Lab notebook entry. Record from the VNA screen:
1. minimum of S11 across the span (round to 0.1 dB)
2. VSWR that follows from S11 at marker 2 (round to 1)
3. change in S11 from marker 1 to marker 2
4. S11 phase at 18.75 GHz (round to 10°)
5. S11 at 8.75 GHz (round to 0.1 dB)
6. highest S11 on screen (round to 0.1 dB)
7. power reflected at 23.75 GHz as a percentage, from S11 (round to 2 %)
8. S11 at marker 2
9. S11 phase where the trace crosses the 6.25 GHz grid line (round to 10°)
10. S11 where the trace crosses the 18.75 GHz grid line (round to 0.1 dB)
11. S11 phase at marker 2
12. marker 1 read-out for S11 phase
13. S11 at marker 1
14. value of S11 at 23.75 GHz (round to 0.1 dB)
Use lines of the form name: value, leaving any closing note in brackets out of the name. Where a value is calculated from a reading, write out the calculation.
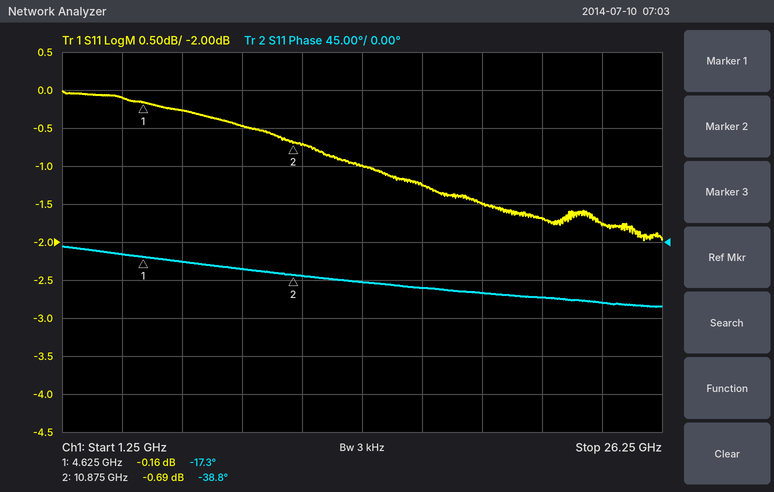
minimum of S11 across the span: -2.0 dB
VSWR that follows from S11 at marker 2: (1 + 0.9236)/(1 − 0.9236) ≈ 25
change in S11 from marker 1 to marker 2: -0.69 − (-0.16) = -0.53 dB
S11 phase at 18.75 GHz: -60°
S11 at 8.75 GHz: -0.5 dB
highest S11 on screen: 0.0 dB
power reflected at 23.75 GHz as a percentage, from S11: 10^(-1.8/10) ≈ 66 %
S11 at marker 2: -0.69 dB
S11 phase where the trace crosses the 6.25 GHz grid line: -20°
S11 where the trace crosses the 18.75 GHz grid line: -1.5 dB
S11 phase at marker 2: -38.8°
marker 1 read-out for S11 phase: -17.3°
S11 at marker 1: -0.16 dB
value of S11 at 23.75 GHz: -1.8 dB
